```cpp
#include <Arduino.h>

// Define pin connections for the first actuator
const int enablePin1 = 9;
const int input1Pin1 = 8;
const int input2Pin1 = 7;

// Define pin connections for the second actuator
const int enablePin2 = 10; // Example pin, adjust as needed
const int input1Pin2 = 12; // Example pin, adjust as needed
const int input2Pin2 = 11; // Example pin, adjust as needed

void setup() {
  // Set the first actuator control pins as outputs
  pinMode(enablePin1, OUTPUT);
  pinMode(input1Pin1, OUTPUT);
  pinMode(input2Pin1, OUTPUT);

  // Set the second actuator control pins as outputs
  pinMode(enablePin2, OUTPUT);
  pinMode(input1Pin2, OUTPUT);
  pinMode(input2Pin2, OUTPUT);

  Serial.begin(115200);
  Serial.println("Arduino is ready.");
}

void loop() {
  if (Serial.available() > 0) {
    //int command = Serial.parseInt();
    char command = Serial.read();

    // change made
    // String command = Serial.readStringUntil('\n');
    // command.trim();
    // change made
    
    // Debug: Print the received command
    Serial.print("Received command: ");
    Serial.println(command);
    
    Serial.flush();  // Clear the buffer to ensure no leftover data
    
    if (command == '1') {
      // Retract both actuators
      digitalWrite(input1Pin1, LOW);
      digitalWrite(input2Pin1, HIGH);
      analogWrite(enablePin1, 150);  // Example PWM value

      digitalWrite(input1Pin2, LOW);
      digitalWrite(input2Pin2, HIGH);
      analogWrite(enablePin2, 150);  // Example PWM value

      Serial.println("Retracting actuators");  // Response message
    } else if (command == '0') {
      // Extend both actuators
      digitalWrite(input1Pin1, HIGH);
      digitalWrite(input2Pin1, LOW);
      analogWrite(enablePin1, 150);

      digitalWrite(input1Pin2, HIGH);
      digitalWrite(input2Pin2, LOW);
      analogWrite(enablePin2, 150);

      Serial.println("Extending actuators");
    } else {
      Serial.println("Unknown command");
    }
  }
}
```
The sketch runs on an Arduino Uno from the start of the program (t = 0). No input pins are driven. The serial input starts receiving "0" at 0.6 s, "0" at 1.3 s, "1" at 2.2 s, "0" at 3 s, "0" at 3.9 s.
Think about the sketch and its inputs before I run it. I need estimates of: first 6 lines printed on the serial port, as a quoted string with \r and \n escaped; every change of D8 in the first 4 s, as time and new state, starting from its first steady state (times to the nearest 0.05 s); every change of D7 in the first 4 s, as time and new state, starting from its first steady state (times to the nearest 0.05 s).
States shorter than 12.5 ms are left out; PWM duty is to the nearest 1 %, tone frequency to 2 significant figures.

"Arduino is ready.\r\nReceived command: 0\r\nExtending actuators\r\nReceived command: 0\r\nExtending actuators\r\nReceived command: 1\r\n"
0 s low; 0.6 s high; 2.2 s low; 3 s high
0 s low; 2.2 s high; 3 s low
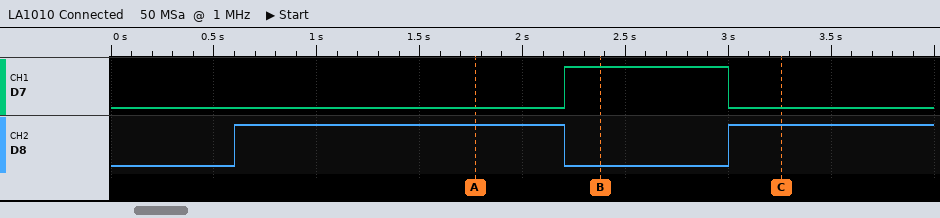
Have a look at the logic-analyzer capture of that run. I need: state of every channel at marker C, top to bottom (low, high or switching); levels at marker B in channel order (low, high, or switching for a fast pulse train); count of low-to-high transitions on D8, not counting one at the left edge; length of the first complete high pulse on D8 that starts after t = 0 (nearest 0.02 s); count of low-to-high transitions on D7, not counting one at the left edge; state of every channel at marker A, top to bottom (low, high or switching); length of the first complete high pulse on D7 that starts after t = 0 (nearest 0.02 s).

D7 low, D8 high
D7 high, D8 low
2
1.60 s
1
D7 low, D8 high
0.80 s
